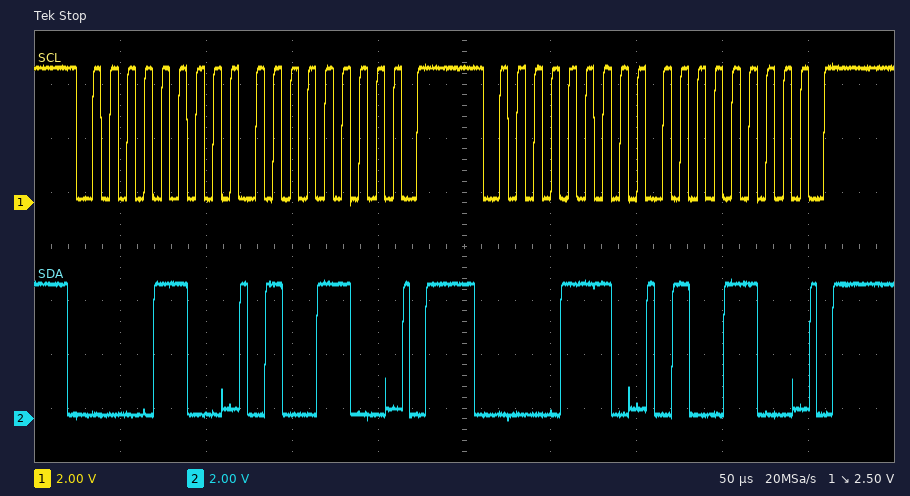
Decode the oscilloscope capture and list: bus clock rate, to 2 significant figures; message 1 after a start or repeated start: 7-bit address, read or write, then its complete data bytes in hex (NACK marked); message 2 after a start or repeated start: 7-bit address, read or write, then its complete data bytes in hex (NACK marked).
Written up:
100 kHz
0x06 write: 4C
0x07 write: 4C
